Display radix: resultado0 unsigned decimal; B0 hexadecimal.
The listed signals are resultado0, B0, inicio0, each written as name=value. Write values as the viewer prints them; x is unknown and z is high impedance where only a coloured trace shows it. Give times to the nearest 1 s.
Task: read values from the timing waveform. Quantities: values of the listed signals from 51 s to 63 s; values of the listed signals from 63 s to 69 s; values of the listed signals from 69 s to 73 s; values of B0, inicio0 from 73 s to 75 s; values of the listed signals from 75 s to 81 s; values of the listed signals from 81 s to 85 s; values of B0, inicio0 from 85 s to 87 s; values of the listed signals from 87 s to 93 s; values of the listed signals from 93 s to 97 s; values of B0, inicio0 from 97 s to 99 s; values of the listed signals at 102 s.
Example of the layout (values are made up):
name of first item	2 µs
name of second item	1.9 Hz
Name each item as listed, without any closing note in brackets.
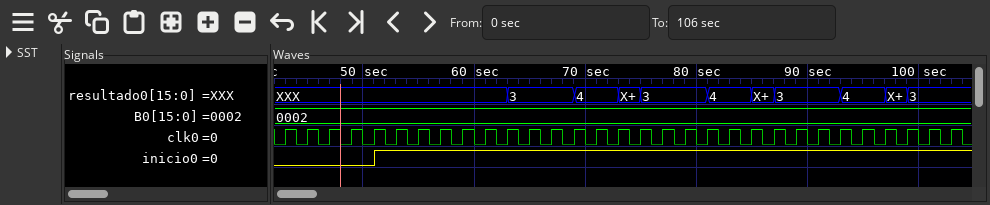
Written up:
values of the listed signals from 51 s to 63 s	resultado0=XXX, B0=0002, inicio0=1
values of the listed signals from 63 s to 69 s	resultado0=3, B0=0002, inicio0=1
values of the listed signals from 69 s to 73 s	resultado0=4, B0=0002, inicio0=1
values of B0, inicio0 from 73 s to 75 s	B0=0002, inicio0=1
values of the listed signals from 75 s to 81 s	resultado0=3, B0=0002, inicio0=1
values of the listed signals from 81 s to 85 s	resultado0=4, B0=0002, inicio0=1
values of B0, inicio0 from 85 s to 87 s	B0=0002, inicio0=1
values of the listed signals from 87 s to 93 s	resultado0=3, B0=0002, inicio0=1
values of the listed signals from 93 s to 97 s	resultado0=4, B0=0002, inicio0=1
values of B0, inicio0 from 97 s to 99 s	B0=0002, inicio0=1
values of the listed signals at 102 s	resultado0=3, B0=0002, inicio0=1
